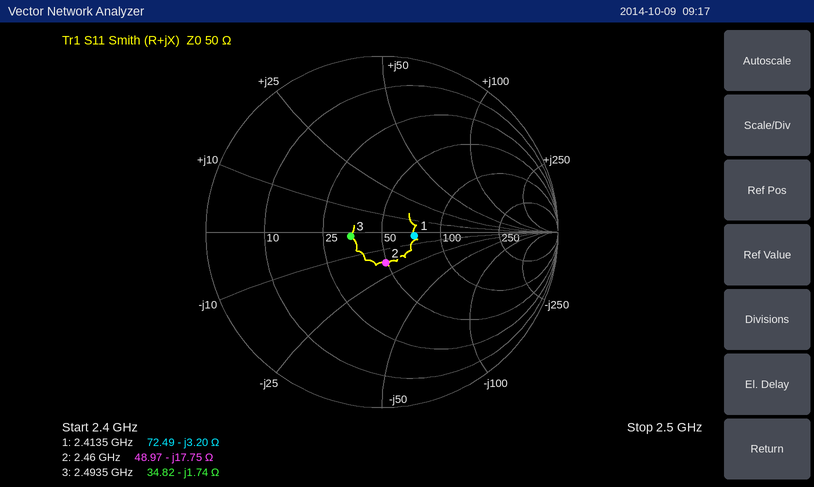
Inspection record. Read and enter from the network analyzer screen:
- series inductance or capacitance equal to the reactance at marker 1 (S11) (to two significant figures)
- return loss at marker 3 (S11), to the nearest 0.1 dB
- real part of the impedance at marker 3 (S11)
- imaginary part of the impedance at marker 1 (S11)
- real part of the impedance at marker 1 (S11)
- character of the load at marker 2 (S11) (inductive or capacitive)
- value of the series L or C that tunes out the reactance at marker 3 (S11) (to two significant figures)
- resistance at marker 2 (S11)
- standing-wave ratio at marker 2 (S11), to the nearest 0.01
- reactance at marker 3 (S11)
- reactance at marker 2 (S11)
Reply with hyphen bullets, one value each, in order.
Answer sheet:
- 21 pF
- 14.9 dB
- 34.82 Ω
- -3.20 Ω
- 72.49 Ω
- capacitive
- 110 pH
- 48.97 Ω
- 1.43
- -1.74 Ω
- -17.75 Ω
